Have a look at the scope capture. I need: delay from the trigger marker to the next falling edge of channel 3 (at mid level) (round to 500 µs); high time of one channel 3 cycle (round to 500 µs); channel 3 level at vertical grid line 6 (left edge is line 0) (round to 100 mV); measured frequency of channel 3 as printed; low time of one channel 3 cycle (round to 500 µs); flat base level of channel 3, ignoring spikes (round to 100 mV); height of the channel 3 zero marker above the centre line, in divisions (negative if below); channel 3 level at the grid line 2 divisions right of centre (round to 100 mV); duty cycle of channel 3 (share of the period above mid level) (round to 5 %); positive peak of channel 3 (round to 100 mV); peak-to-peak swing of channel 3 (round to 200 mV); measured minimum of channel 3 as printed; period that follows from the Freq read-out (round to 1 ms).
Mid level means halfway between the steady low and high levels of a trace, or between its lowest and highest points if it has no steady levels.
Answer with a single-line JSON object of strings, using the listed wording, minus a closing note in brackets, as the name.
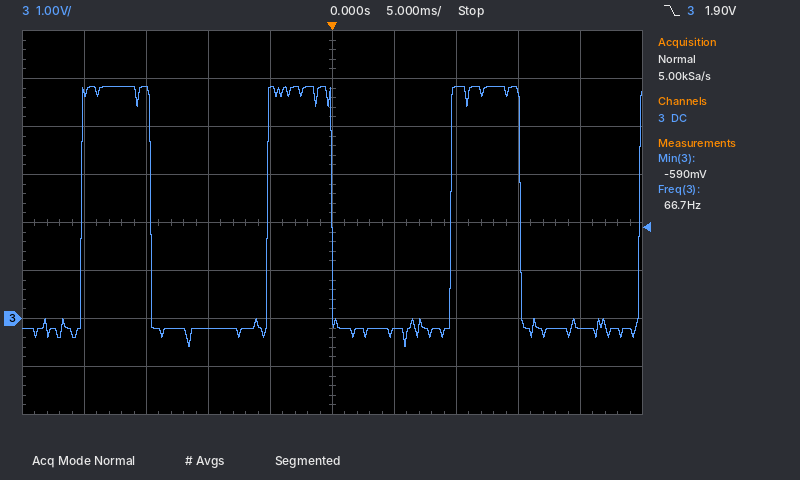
{"delay from the trigger marker to the next falling edge of channel 3 (at mid level)": "15.0 ms", "high time of one channel 3 cycle": "5.5 ms", "channel 3 level at vertical grid line 6 (left edge is line 0)": "-300 mV", "measured frequency of channel 3 as printed": "66.7 Hz", "low time of one channel 3 cycle": "9.5 ms", "flat base level of channel 3, ignoring spikes": "-200 mV", "height of the channel 3 zero marker above the centre line, in divisions": "-2.0 div", "channel 3 level at the grid line 2 divisions right of centre": "4.8 V", "duty cycle of channel 3 (share of the period above mid level)": "35 %", "positive peak of channel 3": "4.8 V", "peak-to-peak swing of channel 3": "5.4 V", "measured minimum of channel 3 as printed": "-590 mV", "period that follows from the Freq read-out": "15 ms"}
